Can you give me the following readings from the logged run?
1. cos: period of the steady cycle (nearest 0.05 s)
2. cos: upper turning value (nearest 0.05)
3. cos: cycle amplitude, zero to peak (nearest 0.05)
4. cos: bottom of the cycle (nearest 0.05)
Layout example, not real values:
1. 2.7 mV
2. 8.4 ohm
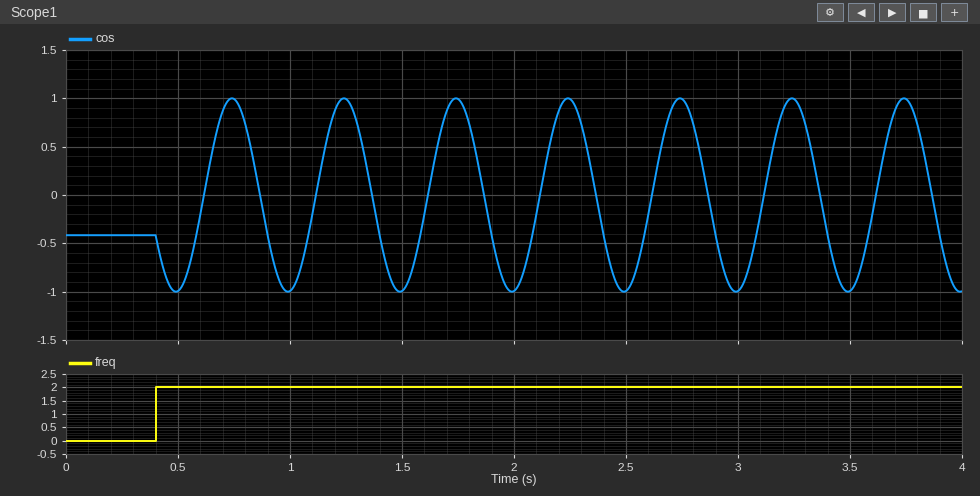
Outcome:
1. 0.50 s
2. 1.00
3. 1.00
4. -1.00
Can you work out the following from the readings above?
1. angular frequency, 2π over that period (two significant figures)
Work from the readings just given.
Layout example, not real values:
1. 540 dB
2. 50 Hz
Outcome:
1. 13 rad/s
